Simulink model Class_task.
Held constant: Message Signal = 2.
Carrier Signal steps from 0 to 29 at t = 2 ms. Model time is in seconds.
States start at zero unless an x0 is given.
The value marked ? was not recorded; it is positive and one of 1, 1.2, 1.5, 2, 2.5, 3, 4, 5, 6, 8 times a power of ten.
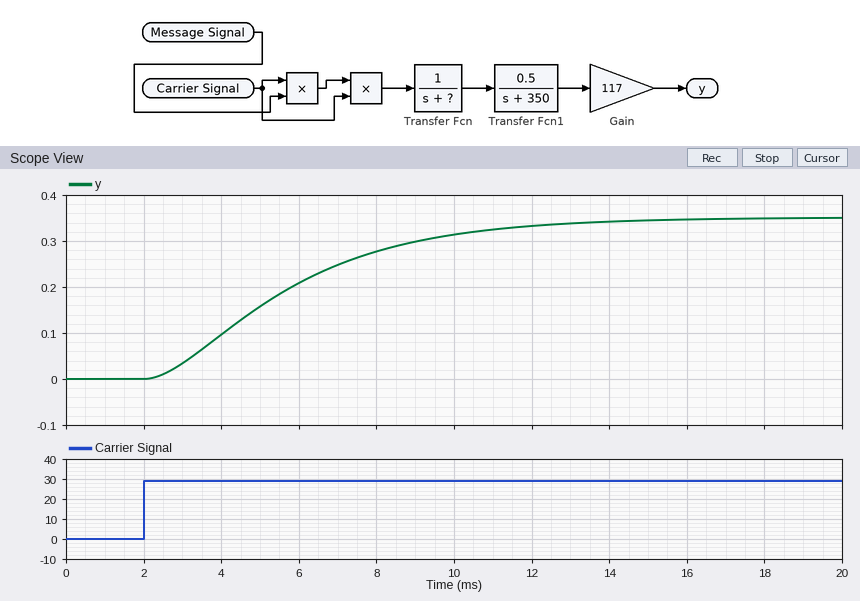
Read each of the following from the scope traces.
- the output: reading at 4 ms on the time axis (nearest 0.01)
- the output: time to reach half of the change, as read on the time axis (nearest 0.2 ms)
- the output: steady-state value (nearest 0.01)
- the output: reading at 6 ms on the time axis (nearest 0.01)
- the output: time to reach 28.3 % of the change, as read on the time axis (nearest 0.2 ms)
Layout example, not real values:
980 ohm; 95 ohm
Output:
0.10; 5.4 ms; 0.35; 0.21; 4.0 ms
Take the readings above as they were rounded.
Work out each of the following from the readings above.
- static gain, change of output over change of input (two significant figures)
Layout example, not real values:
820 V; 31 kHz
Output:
0.012
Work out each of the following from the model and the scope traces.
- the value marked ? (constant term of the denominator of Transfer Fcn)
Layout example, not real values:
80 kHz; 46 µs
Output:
800
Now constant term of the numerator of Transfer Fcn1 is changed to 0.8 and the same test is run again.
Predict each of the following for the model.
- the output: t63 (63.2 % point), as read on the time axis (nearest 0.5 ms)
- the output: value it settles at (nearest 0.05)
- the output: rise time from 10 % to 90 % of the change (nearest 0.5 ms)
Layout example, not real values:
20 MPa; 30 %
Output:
6.5 ms; 0.55; 7.0 ms
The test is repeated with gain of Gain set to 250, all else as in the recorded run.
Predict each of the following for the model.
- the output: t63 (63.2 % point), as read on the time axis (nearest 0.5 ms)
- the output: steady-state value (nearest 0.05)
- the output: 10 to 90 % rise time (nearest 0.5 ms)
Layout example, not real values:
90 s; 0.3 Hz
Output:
6.5 ms; 0.75; 7.0 ms
